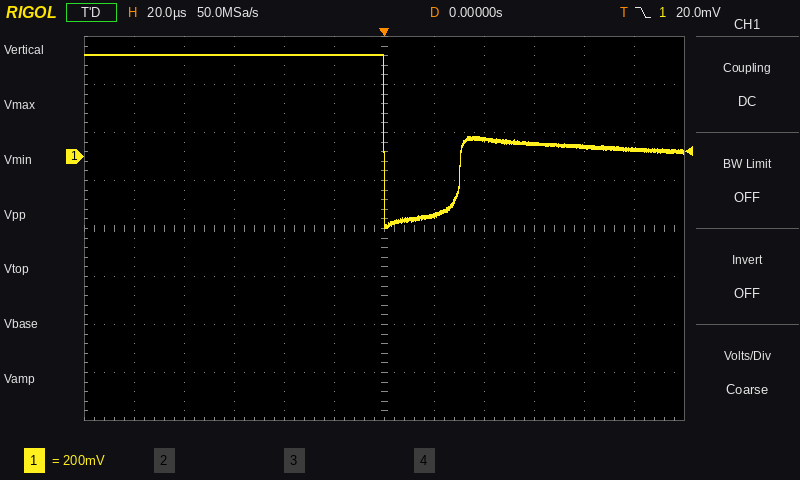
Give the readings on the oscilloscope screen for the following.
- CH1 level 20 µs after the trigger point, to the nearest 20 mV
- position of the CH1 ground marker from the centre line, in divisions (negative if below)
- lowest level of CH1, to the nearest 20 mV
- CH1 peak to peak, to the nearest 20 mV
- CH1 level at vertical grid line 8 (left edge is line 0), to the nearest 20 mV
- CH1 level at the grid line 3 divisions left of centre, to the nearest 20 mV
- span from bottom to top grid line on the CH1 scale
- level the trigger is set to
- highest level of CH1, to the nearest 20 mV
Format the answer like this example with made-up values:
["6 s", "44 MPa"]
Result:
["-240 mV", "+1.5 div", "-300 mV", "720 mV", "80 mV", "420 mV", "1.6 V", "20.0 mV", "420 mV"]
